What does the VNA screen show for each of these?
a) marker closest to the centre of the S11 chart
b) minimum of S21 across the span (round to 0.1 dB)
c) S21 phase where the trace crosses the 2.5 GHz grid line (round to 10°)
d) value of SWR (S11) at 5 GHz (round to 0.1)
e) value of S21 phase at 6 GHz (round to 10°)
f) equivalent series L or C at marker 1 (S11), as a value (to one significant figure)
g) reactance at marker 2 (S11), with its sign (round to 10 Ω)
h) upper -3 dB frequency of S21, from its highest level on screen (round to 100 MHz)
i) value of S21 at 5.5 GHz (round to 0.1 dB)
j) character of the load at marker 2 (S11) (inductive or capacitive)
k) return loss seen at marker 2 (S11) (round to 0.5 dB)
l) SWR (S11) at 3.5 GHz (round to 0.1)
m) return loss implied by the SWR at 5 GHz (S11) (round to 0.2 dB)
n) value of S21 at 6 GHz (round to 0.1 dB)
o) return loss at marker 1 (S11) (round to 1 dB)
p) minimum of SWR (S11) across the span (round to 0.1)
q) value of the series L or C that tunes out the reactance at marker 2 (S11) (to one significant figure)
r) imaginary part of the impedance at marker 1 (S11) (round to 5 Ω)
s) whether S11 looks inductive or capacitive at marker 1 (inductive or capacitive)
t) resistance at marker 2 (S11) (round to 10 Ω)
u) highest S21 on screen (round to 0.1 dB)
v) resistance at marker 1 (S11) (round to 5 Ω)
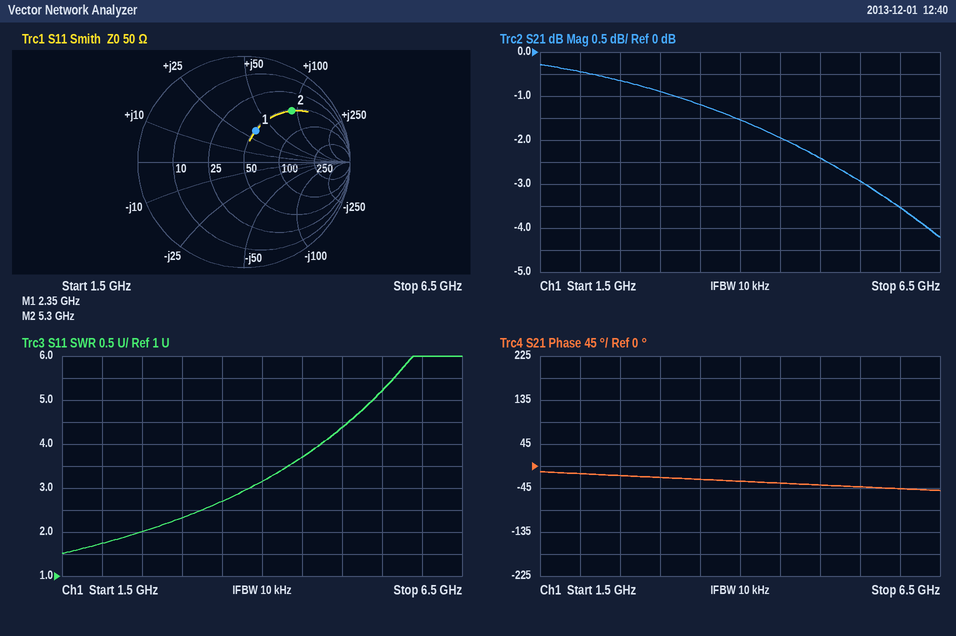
marker 1
-4.2 dB
-20°
4.4
-50°
2 nH
+90 Ω
5.8 GHz
-2.9 dB
inductive
3.5 dB
2.7
4.0 dB
-3.5 dB
10 dB
1.5
300 fF
+35 Ω
inductive
50 Ω
-0.3 dB
50 Ω
